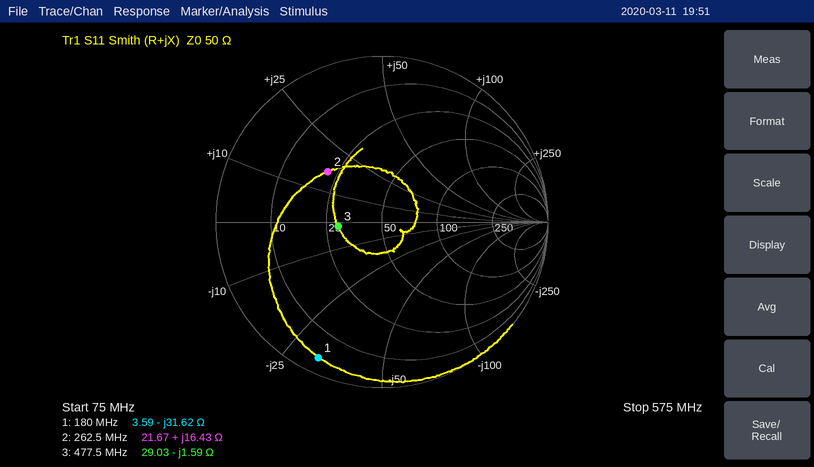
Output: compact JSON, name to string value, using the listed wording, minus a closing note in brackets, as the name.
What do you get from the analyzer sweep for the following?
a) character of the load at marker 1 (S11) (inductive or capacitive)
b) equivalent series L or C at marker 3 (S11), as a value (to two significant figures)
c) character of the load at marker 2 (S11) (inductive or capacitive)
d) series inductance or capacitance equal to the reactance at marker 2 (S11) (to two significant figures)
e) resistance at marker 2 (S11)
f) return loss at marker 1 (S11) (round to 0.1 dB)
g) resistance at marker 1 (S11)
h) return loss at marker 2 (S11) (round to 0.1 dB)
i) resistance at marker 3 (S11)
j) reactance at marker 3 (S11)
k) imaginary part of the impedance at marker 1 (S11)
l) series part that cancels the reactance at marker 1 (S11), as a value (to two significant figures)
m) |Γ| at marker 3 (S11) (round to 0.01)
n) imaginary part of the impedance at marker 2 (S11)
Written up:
{"character of the load at marker 1 (S11)": "capacitive", "equivalent series L or C at marker 3 (S11), as a value": "210 pF", "character of the load at marker 2 (S11)": "inductive", "series inductance or capacitance equal to the reactance at marker 2 (S11)": "10.0 nH", "resistance at marker 2": "21.67 Ω", "return loss at marker 1 (S11)": "0.9 dB", "resistance at marker 1": "3.59 Ω", "return loss at marker 2 (S11)": "7.0 dB", "resistance at marker 3": "29.03 Ω", "reactance at marker 3": "-1.59 Ω", "imaginary part of the impedance at marker 1": "-31.62 Ω", "series part that cancels the reactance at marker 1 (S11), as a value": "28 nH", "|Γ| at marker 3 (S11)": "0.27", "imaginary part of the impedance at marker 2": "+16.43 Ω"}
